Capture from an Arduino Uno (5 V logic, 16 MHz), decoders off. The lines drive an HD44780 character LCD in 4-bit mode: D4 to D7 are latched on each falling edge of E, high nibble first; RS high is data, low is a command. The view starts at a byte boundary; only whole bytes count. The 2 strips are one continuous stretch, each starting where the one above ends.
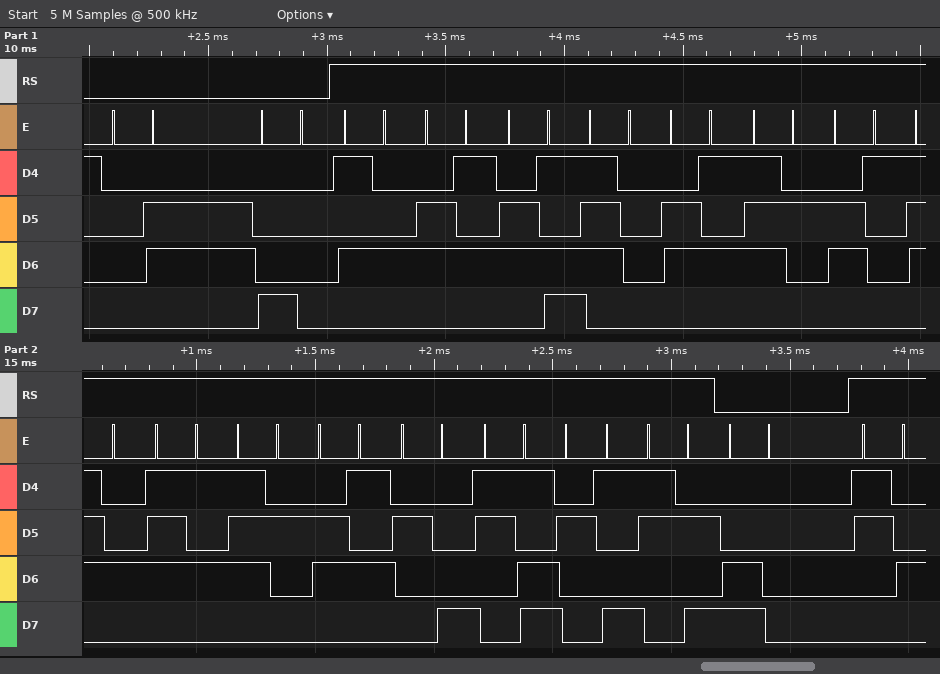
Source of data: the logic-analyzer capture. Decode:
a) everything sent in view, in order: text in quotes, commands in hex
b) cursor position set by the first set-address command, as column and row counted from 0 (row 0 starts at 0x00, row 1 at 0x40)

0x06 0x80 "Temperature(=):" 0xC0 "4"
column 0, row 0
